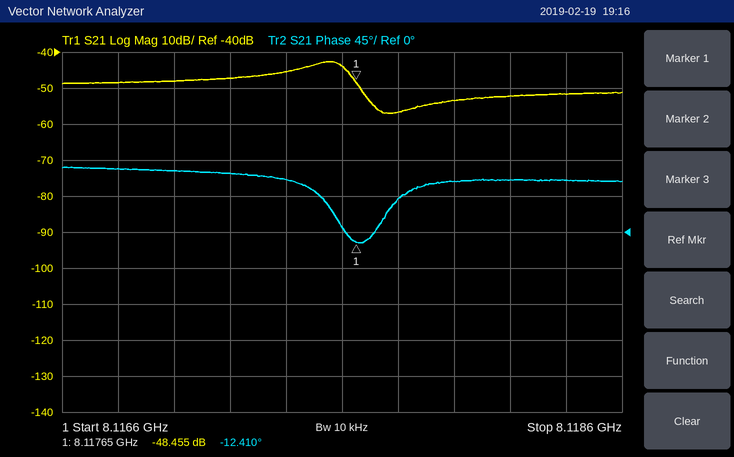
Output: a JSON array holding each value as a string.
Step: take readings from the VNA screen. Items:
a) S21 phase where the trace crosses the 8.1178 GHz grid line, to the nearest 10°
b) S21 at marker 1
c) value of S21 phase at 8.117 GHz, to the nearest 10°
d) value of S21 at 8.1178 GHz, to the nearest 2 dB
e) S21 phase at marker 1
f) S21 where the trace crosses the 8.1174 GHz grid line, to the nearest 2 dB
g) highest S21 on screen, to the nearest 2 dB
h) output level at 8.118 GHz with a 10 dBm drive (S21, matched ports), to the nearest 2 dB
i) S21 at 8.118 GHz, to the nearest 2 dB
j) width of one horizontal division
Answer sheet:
["40°", "-48.455 dB", "80°", "-56 dB", "-12.410°", "-46 dB", "-42 dB", "-44 dBm", "-54 dB", "200 kHz"]
